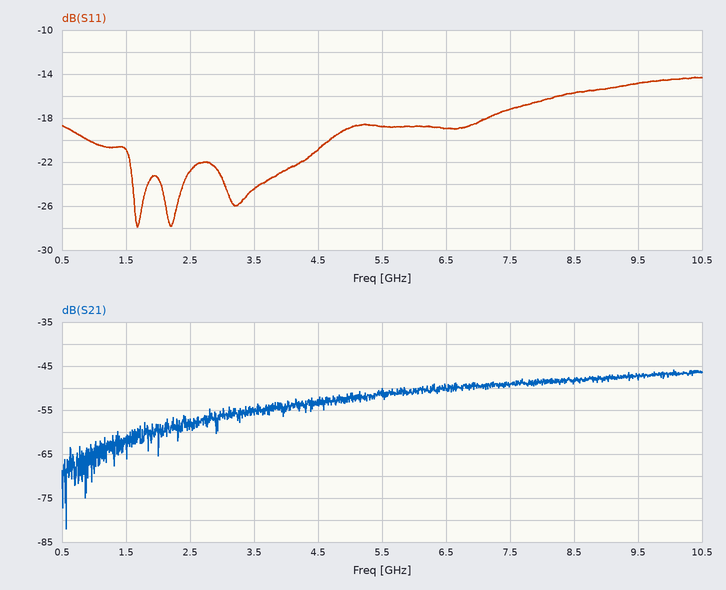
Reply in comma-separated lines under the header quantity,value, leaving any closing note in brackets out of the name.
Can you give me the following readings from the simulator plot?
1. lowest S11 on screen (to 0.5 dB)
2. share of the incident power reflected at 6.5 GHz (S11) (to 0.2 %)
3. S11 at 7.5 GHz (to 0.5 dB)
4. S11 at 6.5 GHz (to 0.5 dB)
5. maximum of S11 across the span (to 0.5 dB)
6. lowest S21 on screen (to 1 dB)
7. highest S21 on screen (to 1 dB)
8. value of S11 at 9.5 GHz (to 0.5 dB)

quantity,value
lowest S11 on screen,-28.0 dB
share of the incident power reflected at 6.5 GHz (S11),1.2 %
S11 at 7.5 GHz,-17.0 dB
S11 at 6.5 GHz,-19.0 dB
maximum of S11 across the span,-14.5 dB
lowest S21 on screen,-82 dB
highest S21 on screen,-46 dB
value of S11 at 9.5 GHz,-15.0 dB
